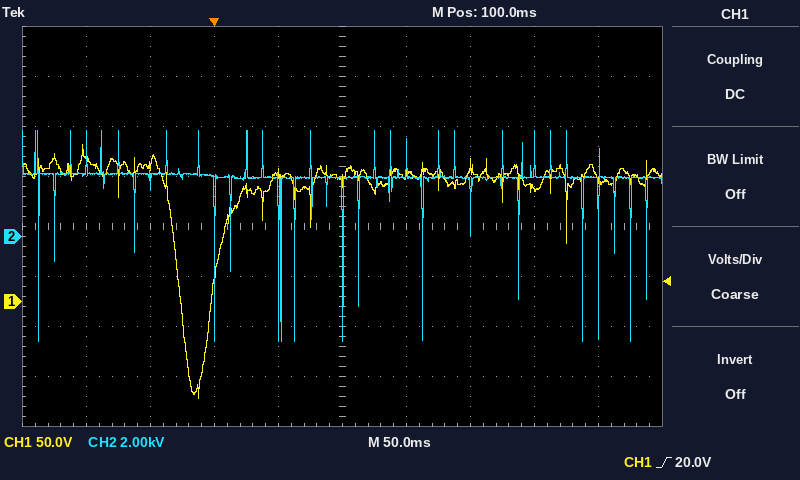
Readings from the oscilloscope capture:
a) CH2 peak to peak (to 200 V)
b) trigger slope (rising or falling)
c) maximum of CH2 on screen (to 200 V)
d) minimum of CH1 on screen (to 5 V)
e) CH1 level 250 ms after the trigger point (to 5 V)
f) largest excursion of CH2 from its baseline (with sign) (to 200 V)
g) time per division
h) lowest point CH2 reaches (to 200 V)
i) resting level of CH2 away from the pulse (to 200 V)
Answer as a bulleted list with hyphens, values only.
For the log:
- 8.4 kV
- rising
- 4.2 kV
- -95 V
- 115 V
- -6.6 kV
- 50 ms
- -4.2 kV
- 2.4 kV
